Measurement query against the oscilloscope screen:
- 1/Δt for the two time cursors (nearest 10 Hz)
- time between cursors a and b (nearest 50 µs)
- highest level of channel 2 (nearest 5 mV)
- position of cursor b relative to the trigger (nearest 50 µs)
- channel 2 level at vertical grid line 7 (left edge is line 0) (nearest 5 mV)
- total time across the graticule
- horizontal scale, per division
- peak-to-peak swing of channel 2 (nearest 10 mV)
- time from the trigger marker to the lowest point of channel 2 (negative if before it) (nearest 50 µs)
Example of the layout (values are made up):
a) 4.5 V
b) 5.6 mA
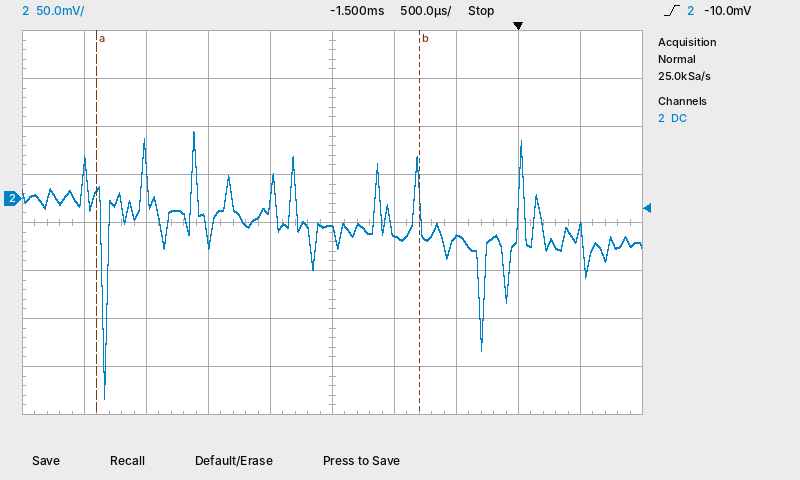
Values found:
a) 380 Hz
b) 2.60 ms
c) 70 mV
d) -800 µs
e) -40 mV
f) 5 ms
g) 500 µs
h) 280 mV
i) -3.35 ms
